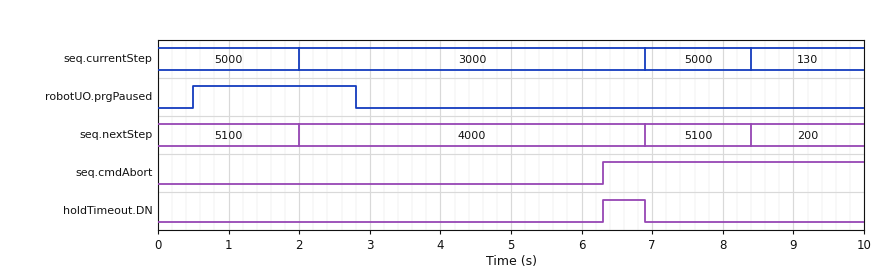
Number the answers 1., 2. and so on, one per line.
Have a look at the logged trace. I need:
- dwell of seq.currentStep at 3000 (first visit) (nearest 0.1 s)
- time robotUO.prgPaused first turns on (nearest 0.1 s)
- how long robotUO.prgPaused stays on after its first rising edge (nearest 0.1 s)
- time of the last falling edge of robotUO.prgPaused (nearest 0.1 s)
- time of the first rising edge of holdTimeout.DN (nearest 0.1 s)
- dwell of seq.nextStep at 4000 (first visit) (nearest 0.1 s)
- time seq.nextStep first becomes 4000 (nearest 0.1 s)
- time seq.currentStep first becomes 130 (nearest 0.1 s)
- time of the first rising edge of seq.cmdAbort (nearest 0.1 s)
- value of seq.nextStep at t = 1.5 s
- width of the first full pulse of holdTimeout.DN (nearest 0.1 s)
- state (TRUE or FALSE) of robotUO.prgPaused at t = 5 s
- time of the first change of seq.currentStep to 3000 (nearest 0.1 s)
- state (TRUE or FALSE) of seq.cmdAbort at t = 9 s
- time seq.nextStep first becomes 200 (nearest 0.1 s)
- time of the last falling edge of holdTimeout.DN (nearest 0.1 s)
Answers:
1. 4.9 s
2. 0.5 s
3. 2.3 s
4. 2.8 s
5. 6.3 s
6. 4.9 s
7. 2.0 s
8. 8.4 s
9. 6.3 s
10. 5100
11. 0.6 s
12. FALSE
13. 2.0 s
14. TRUE
15. 8.4 s
16. 6.9 s
